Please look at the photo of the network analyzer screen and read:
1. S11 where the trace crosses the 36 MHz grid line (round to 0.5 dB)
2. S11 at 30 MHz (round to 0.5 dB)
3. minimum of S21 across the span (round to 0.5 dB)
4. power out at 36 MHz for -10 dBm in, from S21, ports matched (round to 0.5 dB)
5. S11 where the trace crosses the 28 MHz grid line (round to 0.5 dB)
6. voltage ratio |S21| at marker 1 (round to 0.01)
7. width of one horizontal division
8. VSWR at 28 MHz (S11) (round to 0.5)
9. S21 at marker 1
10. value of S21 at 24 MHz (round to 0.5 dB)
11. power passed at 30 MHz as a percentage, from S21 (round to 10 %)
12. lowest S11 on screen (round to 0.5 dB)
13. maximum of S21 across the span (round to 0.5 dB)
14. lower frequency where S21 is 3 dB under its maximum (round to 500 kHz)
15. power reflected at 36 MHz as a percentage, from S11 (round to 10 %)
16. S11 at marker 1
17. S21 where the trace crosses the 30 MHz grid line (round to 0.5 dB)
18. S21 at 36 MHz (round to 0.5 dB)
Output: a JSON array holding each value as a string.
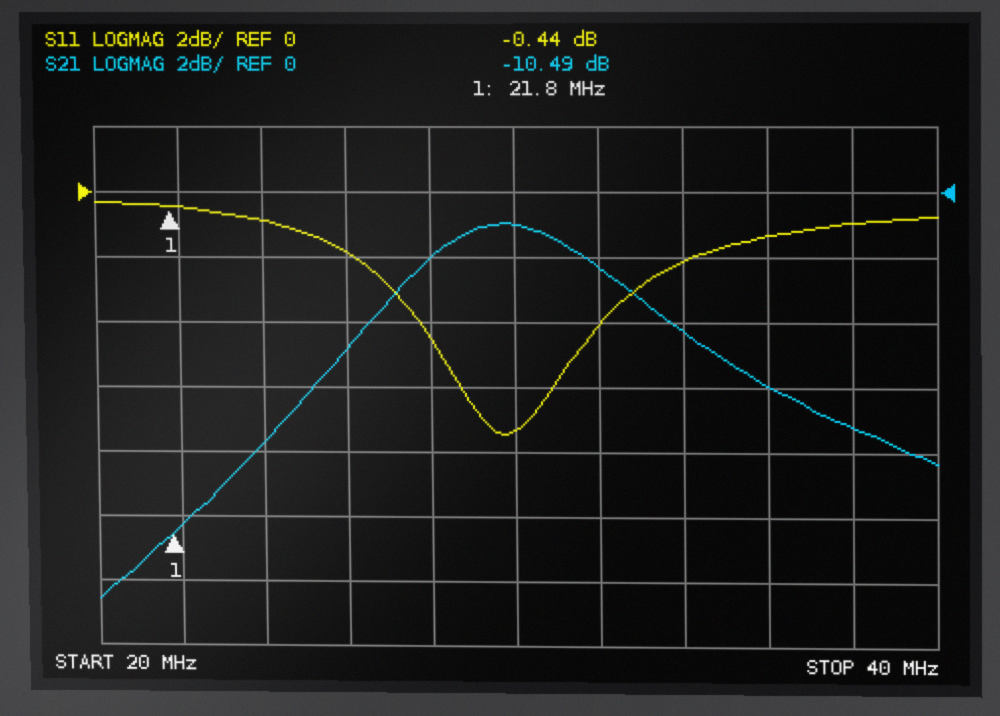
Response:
["-1.5 dB", "-7.5 dB", "-12.5 dB", "-16.0 dBm", "-4.5 dB", "0.30", "2 MHz", "4.0", "-10.49 dB", "-7.5 dB", "80 %", "-7.5 dB", "-1.0 dB", "26.5 MHz", "70 %", "-0.44 dB", "-1.0 dB", "-6.0 dB"]
